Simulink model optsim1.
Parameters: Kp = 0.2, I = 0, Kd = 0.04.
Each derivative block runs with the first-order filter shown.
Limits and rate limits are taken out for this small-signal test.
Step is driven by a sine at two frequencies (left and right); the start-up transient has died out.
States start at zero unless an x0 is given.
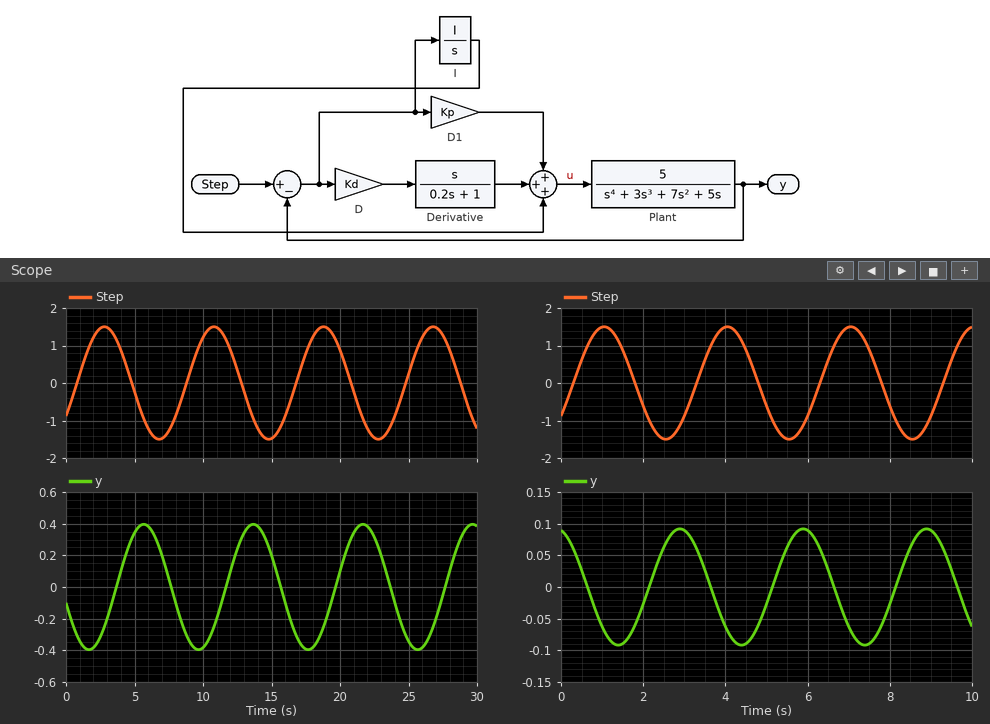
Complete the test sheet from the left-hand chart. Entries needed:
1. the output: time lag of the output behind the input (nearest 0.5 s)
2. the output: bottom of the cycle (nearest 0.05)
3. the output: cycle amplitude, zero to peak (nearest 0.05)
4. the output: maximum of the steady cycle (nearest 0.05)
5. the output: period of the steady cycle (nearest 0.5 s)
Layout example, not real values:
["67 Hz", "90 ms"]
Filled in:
["3.0 s", "-0.40", "0.40", "0.40", "8.0 s"]
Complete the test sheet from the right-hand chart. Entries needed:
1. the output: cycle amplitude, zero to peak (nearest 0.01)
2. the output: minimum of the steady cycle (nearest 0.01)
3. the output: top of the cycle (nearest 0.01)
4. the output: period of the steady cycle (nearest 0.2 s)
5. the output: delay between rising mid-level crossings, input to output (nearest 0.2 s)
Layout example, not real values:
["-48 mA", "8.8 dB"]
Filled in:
["0.09", "-0.09", "0.09", "3.0 s", "1.8 s"]
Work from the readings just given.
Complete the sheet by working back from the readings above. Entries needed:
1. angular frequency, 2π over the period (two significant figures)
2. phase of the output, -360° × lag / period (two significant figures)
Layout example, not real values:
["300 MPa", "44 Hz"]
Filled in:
["2.1 rad/s", "-220°"]
